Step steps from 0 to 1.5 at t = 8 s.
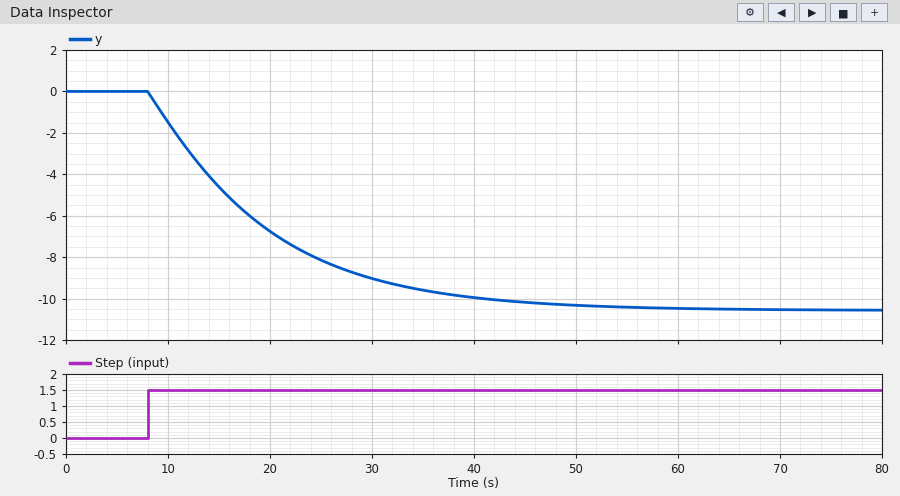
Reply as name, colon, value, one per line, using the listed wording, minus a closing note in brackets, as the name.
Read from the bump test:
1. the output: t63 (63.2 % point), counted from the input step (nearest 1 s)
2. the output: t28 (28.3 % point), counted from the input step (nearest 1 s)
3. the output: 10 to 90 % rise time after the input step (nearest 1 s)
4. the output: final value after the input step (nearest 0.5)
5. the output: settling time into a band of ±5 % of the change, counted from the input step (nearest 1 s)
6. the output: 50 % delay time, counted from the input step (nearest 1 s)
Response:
the output: t63 (63.2 % point), counted from the input step: 12 s
the output: t28 (28.3 % point), counted from the input step: 4 s
the output: 10 to 90 % rise time after the input step: 25 s
the output: final value after the input step: -10.5
the output: settling time into a band of ±5 % of the change, counted from the input step: 34 s
the output: 50 % delay time, counted from the input step: 8 s
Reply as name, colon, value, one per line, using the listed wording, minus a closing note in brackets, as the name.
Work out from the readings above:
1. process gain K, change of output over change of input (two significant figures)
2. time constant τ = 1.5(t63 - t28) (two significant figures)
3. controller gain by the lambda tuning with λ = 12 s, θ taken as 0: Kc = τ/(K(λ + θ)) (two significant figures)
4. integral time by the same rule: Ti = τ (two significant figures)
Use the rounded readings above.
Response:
process gain K, change of output over change of input: -7.0
time constant τ = 1.5(t63 - t28): 12 s
controller gain by the lambda tuning with λ = 12 s, θ taken as 0: Kc = τ/(K(λ + θ)): -0.14
integral time by the same rule: Ti = τ: 12 s
